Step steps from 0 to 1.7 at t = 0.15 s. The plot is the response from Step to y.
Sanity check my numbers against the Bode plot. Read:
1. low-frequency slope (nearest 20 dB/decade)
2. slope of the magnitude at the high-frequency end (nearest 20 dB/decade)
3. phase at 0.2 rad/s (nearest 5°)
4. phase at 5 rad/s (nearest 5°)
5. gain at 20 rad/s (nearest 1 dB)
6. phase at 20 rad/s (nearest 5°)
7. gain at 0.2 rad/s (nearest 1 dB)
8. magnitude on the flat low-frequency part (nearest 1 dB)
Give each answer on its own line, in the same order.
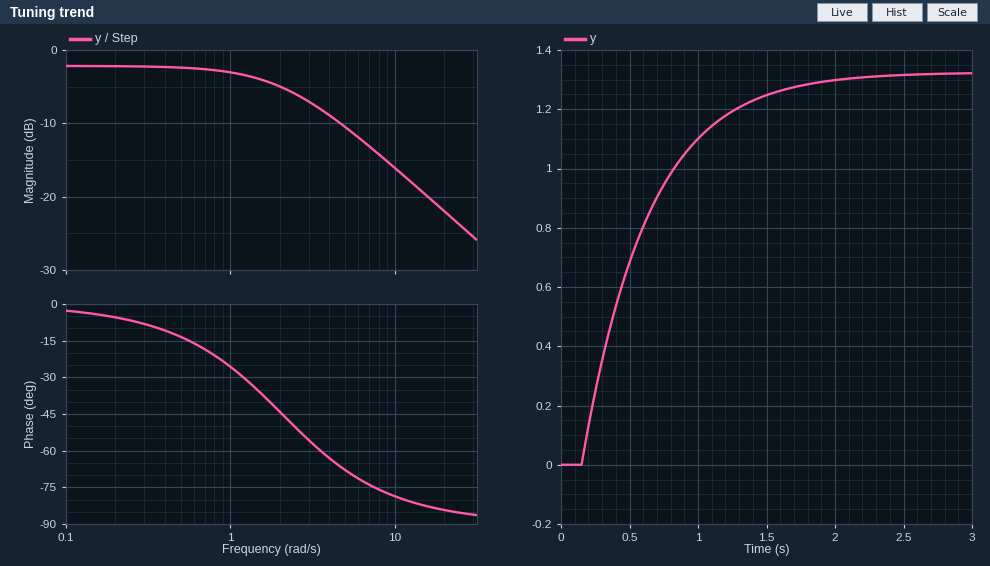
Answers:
0 dB/decade
-20 dB/decade
-5°
-70°
-22 dB
-85°
-2 dB
-2 dB
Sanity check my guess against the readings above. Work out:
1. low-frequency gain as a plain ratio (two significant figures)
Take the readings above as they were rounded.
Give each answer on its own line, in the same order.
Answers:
0.79
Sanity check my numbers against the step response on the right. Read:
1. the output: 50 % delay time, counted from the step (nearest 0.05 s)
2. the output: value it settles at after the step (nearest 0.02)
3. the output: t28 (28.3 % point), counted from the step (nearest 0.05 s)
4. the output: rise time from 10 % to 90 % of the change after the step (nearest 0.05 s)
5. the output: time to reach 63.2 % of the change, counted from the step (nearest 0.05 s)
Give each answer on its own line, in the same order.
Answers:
0.35 s
1.32
0.15 s
1.05 s
0.50 s
